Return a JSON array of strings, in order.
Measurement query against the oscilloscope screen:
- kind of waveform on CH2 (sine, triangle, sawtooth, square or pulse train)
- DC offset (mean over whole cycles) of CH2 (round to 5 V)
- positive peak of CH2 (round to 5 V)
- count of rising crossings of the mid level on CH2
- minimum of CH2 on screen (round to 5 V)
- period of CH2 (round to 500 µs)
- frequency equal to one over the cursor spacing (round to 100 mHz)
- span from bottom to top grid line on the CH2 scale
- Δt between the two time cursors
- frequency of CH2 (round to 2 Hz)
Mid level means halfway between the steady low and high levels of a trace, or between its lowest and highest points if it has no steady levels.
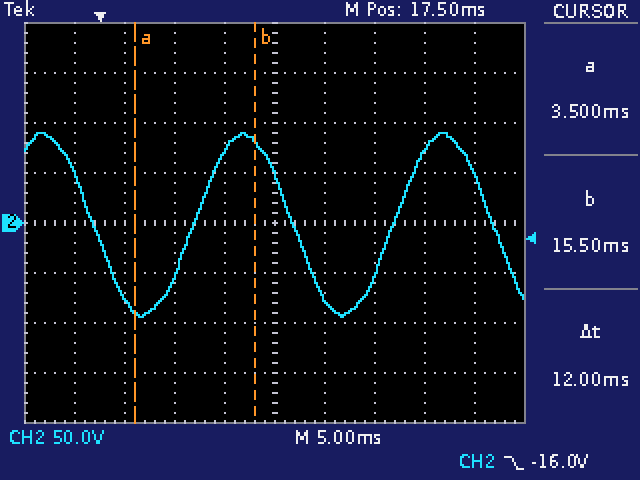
["sine", "0 V", "90 V", "2", "-95 V", "20.0 ms", "83.3 Hz", "400 V", "12 ms", "50 Hz"]
